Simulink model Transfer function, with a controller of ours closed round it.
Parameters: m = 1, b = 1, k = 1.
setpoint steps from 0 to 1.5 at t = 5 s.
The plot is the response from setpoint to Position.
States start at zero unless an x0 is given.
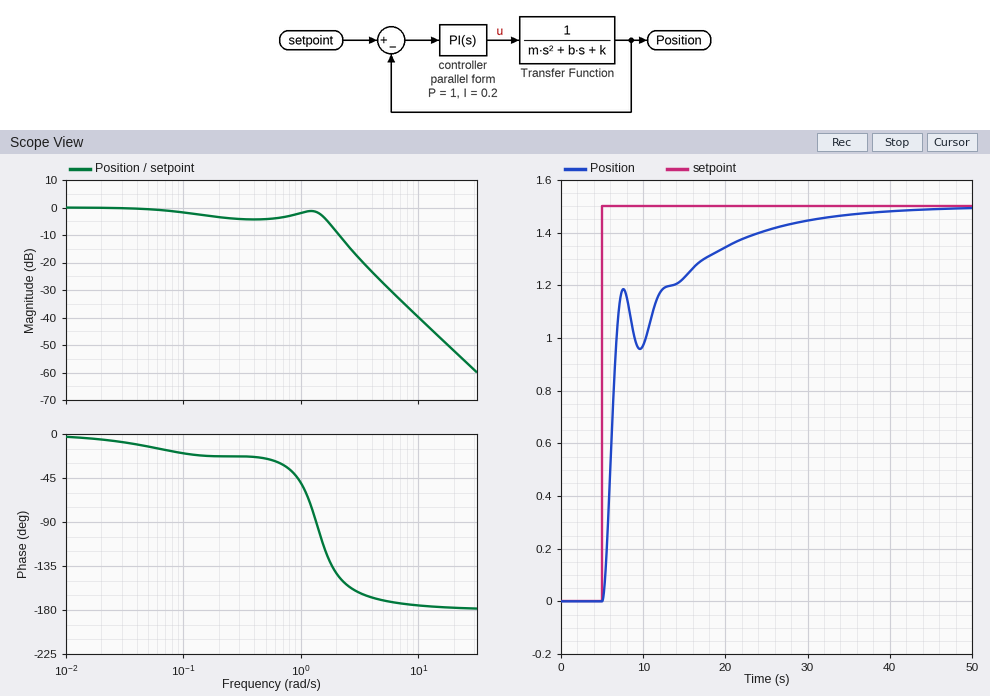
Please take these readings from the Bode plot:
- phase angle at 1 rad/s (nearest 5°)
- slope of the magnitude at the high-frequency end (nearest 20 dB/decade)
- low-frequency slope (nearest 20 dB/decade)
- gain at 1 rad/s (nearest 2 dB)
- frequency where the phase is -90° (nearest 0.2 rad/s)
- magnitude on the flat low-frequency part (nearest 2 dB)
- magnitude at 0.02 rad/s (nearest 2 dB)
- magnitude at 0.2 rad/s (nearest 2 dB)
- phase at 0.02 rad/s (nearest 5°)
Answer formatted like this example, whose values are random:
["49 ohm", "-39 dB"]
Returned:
["-50°", "-40 dB/decade", "0 dB/decade", "-2 dB", "1.4 rad/s", "0 dB", "0 dB", "-4 dB", "-5°"]
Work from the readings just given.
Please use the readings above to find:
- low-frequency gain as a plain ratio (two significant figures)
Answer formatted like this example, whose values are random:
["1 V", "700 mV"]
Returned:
["1.0"]
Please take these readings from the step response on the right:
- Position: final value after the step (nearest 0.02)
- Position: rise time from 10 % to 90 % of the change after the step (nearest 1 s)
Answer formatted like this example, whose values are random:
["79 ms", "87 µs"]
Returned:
["1.50", "15 s"]
